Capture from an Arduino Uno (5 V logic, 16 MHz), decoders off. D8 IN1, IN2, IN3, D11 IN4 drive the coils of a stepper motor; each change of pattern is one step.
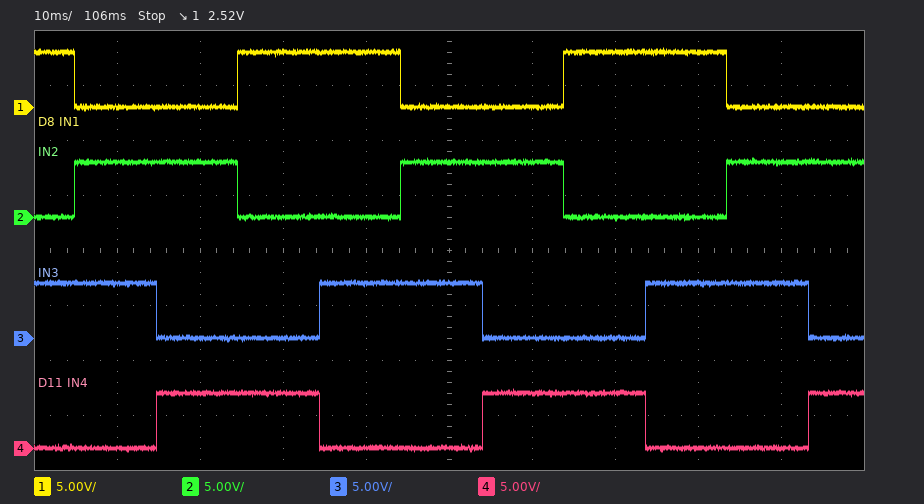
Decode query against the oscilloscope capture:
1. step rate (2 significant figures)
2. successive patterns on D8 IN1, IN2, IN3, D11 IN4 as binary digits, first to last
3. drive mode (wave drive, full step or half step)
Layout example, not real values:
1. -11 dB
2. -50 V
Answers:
1. 100 steps/s
2. 1010 0110 0101 1001 1010 0110 0101 1001 1010 0110 0101
3. full step
